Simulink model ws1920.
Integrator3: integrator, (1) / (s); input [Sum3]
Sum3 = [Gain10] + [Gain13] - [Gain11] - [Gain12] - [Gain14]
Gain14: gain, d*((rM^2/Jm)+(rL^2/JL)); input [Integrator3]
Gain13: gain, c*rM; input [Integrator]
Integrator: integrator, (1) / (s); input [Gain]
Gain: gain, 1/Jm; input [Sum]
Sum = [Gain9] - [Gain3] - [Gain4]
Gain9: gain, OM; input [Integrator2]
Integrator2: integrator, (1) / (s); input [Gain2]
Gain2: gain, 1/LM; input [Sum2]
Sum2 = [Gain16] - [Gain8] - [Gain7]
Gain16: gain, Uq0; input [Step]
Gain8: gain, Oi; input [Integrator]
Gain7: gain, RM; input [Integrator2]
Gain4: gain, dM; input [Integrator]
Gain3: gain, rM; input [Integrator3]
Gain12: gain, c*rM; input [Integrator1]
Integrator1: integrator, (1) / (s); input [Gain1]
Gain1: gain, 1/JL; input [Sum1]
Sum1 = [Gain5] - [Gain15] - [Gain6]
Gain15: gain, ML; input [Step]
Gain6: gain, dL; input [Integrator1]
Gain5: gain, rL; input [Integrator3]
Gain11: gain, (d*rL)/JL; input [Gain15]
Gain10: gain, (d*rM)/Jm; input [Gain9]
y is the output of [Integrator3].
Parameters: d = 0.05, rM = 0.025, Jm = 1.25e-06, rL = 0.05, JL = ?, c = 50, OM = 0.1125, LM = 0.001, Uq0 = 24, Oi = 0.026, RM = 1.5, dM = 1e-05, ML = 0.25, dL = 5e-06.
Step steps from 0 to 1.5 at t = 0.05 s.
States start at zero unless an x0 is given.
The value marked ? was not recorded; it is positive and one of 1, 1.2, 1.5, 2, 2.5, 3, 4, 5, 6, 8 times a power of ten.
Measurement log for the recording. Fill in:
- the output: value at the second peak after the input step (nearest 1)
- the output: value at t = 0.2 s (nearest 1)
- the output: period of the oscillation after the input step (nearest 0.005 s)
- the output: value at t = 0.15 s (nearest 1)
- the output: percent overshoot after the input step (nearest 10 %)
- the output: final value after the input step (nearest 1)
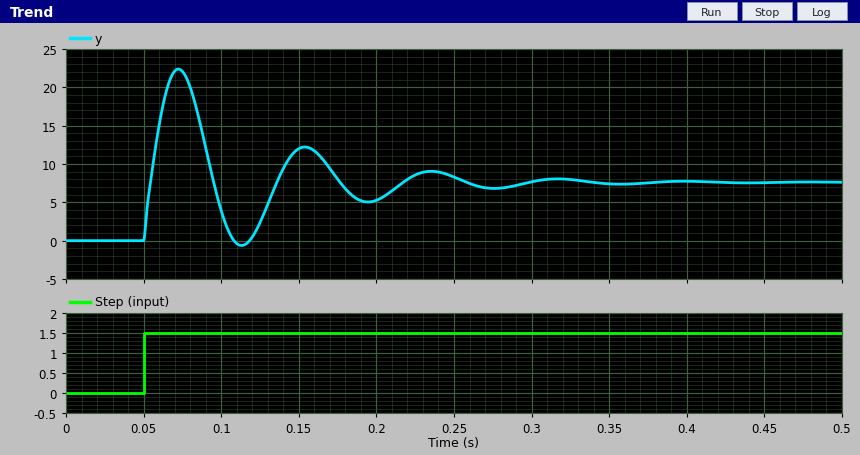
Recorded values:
12
5
0.080 s
12
190 %
8
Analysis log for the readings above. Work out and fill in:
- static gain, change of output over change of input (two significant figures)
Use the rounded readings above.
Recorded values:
5.3
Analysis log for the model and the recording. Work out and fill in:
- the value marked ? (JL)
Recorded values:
1e-05
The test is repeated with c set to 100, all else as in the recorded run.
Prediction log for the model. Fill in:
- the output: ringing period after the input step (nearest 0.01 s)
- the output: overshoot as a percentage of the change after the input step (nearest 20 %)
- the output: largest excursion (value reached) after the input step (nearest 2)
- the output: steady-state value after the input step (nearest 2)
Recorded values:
0.06 s
280 %
28
8
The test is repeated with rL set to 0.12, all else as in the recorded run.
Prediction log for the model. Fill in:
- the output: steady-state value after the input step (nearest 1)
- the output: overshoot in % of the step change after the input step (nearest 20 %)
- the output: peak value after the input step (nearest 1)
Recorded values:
3
200 %
10
